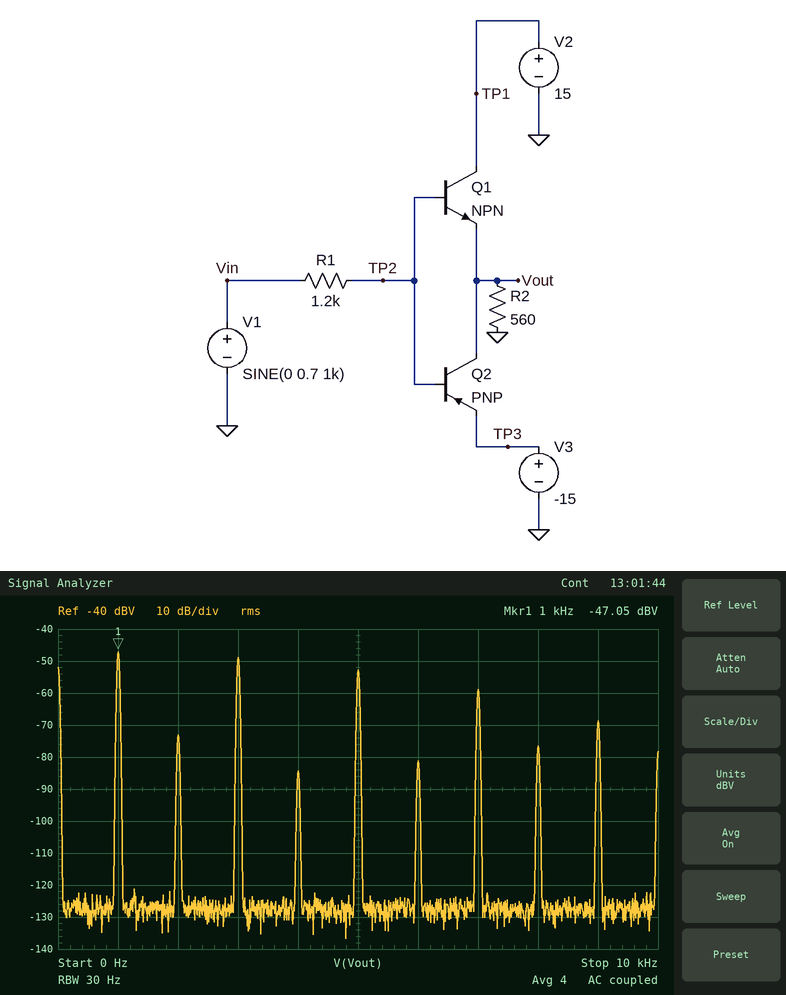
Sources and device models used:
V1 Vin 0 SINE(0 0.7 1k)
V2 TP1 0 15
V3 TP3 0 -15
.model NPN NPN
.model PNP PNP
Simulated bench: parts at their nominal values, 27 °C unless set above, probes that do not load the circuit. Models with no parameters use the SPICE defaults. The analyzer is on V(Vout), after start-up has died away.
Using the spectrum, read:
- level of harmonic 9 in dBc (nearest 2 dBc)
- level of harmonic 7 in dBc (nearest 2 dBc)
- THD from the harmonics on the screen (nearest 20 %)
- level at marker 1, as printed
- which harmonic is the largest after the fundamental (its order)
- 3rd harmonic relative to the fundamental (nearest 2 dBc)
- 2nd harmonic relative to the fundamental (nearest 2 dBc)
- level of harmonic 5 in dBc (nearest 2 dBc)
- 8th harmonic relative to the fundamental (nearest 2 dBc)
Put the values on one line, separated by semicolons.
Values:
-22 dBc; -12 dBc; 100 %; -47.05 dBV; 3; -2 dBc; -26 dBc; -6 dBc; -30 dBc
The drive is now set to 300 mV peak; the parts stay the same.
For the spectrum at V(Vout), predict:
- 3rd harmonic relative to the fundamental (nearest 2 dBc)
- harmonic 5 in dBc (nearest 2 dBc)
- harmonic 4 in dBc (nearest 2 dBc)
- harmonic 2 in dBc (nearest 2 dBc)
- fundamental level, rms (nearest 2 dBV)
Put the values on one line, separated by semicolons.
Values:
-4 dBc; -10 dBc; -10 dBc; -10 dBc; -170 dBV
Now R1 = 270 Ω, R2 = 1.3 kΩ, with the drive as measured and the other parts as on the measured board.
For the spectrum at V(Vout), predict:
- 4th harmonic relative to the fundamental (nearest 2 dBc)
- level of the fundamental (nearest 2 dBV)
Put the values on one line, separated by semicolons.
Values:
-22 dBc; -42 dBV
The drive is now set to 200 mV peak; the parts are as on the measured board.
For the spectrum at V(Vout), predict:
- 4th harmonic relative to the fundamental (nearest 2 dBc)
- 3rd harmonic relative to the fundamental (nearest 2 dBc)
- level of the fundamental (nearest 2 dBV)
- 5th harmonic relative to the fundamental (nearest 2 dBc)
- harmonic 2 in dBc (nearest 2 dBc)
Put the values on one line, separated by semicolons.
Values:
0 dBc; 0 dBc; -180 dBV; 0 dBc; 0 dBc
